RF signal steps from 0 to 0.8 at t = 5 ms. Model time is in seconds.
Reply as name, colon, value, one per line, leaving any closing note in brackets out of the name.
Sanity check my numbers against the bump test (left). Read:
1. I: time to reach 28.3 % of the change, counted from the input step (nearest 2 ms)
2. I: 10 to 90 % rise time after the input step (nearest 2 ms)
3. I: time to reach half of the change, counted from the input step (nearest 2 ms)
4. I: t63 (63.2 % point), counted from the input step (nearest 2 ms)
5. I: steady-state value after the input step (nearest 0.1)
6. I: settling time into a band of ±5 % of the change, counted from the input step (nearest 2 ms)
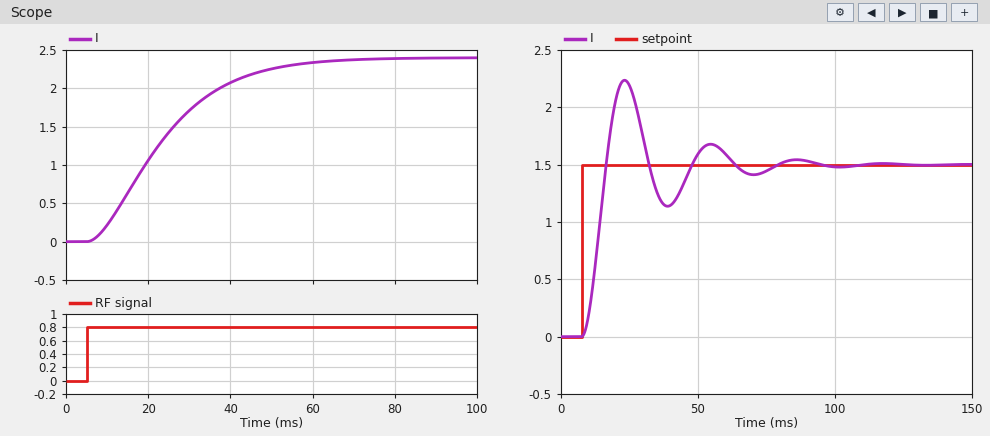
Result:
I: time to reach 28.3 % of the change, counted from the input step: 10 ms
I: 10 to 90 % rise time after the input step: 34 ms
I: time to reach half of the change, counted from the input step: 16 ms
I: t63 (63.2 % point), counted from the input step: 22 ms
I: steady-state value after the input step: 2.4
I: settling time into a band of ±5 % of the change, counted from the input step: 48 ms
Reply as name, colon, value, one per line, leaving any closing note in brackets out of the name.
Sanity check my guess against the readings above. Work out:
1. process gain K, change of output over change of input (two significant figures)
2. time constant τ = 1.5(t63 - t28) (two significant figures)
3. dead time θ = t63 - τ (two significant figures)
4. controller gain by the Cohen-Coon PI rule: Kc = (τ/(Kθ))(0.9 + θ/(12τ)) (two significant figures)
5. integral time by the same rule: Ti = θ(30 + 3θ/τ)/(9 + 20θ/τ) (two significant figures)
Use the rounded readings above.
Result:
process gain K, change of output over change of input: 3.0
time constant τ = 1.5(t63 - t28): 18 ms
dead time θ = t63 - τ: 4.0 ms
controller gain by the Cohen-Coon PI rule: Kc = (τ/(Kθ))(0.9 + θ/(12τ)): 1.4
integral time by the same rule: Ti = θ(30 + 3θ/τ)/(9 + 20θ/τ): 9.1 ms
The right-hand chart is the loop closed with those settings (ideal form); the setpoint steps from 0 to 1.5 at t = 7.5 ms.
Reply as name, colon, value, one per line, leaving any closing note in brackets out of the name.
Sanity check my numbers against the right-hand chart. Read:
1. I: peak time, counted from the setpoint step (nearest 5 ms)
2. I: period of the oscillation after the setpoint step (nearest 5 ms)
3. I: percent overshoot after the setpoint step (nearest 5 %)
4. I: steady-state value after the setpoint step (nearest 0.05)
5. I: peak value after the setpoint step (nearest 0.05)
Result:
I: peak time, counted from the setpoint step: 15 ms
I: period of the oscillation after the setpoint step: 30 ms
I: percent overshoot after the setpoint step: 50 %
I: steady-state value after the setpoint step: 1.50
I: peak value after the setpoint step: 2.25
